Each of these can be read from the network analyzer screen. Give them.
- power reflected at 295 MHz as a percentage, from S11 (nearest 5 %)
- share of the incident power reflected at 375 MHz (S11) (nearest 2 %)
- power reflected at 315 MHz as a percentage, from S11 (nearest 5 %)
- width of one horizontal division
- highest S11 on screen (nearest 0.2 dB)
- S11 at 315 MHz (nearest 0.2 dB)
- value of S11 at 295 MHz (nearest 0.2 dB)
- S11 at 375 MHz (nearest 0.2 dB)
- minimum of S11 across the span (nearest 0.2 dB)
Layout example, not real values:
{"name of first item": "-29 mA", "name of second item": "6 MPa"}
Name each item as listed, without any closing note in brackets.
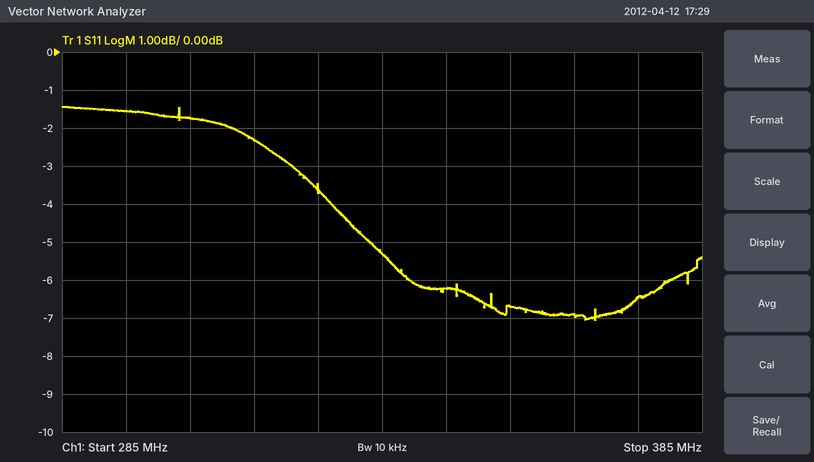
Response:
{"power reflected at 295 MHz as a percentage, from S11": "70 %", "share of the incident power reflected at 375 MHz (S11)": "22 %", "power reflected at 315 MHz as a percentage, from S11": "60 %", "width of one horizontal division": "10 MHz", "highest S11 on screen": "-1.4 dB", "S11 at 315 MHz": "-2.4 dB", "value of S11 at 295 MHz": "-1.6 dB", "S11 at 375 MHz": "-6.4 dB", "minimum of S11 across the span": "-7.0 dB"}
